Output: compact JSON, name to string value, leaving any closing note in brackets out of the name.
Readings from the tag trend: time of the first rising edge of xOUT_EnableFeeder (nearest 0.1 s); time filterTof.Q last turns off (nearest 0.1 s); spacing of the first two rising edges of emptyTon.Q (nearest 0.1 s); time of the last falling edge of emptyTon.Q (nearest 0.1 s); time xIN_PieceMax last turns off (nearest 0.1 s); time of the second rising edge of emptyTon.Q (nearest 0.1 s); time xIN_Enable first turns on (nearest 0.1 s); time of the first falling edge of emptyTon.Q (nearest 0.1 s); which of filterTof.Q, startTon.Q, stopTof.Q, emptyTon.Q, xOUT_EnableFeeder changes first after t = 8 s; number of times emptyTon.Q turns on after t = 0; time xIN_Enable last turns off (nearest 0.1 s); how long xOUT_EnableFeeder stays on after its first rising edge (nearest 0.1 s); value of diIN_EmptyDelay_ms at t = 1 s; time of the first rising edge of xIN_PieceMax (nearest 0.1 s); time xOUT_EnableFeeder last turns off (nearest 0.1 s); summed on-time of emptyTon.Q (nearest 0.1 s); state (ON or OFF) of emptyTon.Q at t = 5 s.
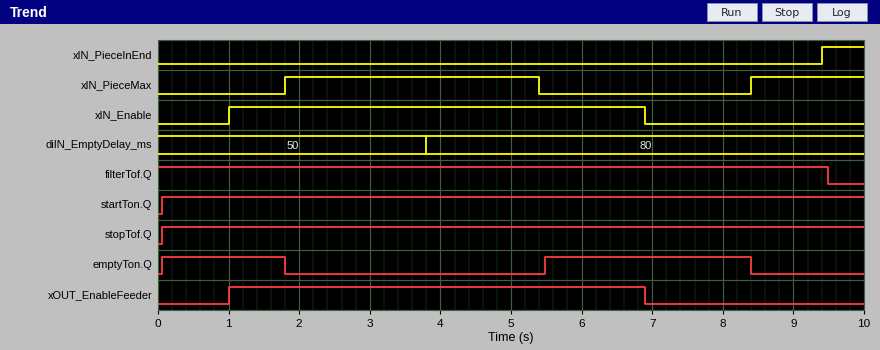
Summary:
{"time of the first rising edge of xOUT_EnableFeeder": "1.0 s", "time filterTof.Q last turns off": "9.5 s", "spacing of the first two rising edges of emptyTon.Q": "5.4 s", "time of the last falling edge of emptyTon.Q": "8.4 s", "time xIN_PieceMax last turns off": "5.4 s", "time of the second rising edge of emptyTon.Q": "5.5 s", "time xIN_Enable first turns on": "1.0 s", "time of the first falling edge of emptyTon.Q": "1.8 s", "which of filterTof.Q, startTon.Q, stopTof.Q, emptyTon.Q, xOUT_EnableFeeder changes first after t = 8 s": "emptyTon.Q", "number of times emptyTon.Q turns on after t = 0": "2", "time xIN_Enable last turns off": "6.9 s", "how long xOUT_EnableFeeder stays on after its first rising edge": "5.9 s", "value of diIN_EmptyDelay_ms at t = 1 s": "50", "time of the first rising edge of xIN_PieceMax": "1.8 s", "time xOUT_EnableFeeder last turns off": "6.9 s", "summed on-time of emptyTon.Q": "4.7 s", "state (ON or OFF) of emptyTon.Q at t = 5 s": "OFF"}
